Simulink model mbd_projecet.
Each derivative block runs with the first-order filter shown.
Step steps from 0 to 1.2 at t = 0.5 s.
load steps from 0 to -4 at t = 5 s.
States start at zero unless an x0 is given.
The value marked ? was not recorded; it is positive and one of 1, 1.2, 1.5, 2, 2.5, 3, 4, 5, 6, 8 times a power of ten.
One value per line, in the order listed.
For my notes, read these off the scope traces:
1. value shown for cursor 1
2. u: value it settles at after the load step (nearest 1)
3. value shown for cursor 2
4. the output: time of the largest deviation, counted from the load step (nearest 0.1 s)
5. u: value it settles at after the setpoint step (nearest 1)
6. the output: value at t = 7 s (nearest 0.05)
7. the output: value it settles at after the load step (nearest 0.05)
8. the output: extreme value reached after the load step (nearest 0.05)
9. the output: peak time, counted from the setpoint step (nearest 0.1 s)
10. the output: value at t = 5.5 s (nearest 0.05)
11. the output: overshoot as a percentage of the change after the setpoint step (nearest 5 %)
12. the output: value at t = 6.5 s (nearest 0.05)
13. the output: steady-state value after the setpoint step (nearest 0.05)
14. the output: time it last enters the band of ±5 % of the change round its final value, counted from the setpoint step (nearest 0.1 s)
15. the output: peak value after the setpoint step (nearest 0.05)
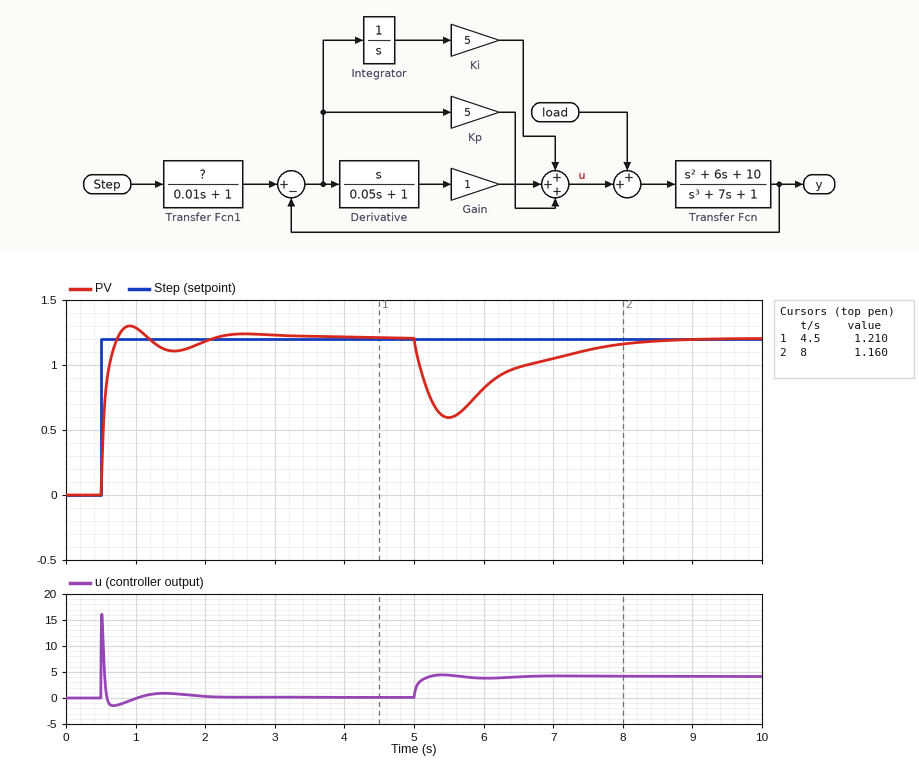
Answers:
1.210
4
1.160
0.5 s
0
1.05
1.20
0.60
0.4 s
0.60
10 %
1.00
1.20
1.3 s
1.30
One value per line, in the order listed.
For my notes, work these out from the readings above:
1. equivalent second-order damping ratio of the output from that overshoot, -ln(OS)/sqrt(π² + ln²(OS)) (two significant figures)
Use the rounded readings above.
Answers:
0.59
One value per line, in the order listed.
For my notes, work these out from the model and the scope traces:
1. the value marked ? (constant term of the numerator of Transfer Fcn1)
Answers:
1
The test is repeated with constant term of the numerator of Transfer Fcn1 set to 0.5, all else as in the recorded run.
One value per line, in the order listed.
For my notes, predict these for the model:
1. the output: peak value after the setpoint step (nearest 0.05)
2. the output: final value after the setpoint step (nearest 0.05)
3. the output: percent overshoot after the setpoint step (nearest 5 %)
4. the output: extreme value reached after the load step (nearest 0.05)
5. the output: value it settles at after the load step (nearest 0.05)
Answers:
0.65
0.60
10 %
0.00
0.60
